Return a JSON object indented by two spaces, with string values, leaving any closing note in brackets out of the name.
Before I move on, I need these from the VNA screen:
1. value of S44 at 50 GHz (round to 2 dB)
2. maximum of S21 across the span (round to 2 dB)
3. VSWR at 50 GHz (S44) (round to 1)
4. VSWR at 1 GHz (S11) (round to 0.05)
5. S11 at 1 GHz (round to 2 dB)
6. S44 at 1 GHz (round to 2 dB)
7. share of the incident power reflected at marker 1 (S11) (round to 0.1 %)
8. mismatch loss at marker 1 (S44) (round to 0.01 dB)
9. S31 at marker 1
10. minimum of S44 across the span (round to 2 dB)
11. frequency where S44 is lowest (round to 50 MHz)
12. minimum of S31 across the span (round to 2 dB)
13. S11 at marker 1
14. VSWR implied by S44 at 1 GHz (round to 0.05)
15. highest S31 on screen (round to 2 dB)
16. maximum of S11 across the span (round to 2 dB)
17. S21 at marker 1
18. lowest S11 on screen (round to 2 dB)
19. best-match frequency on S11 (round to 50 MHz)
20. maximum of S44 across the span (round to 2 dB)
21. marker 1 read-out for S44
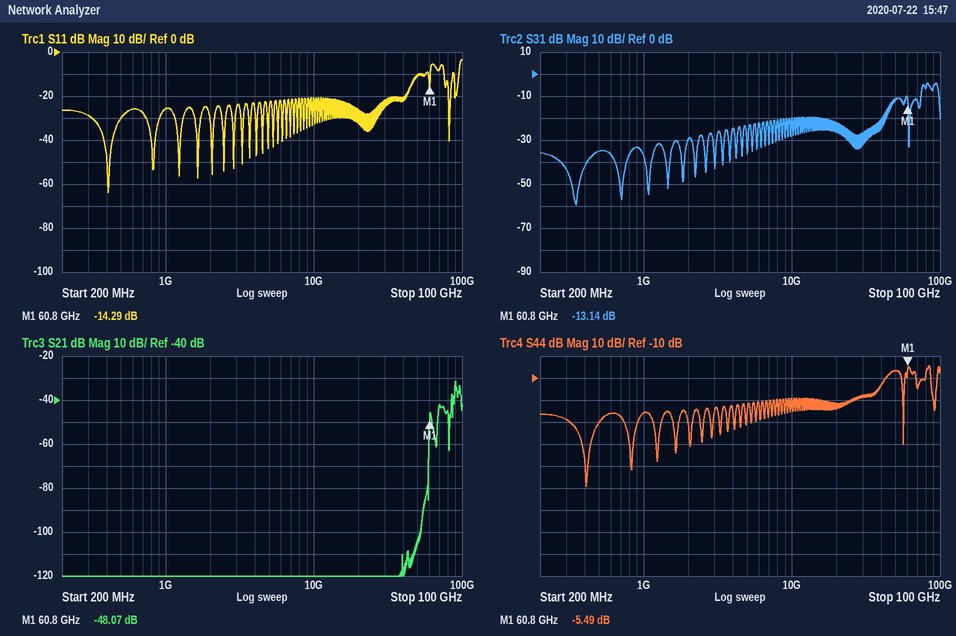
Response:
{
  "value of S44 at 50 GHz": "-6 dB",
  "maximum of S21 across the span": "-32 dB",
  "VSWR at 50 GHz (S44)": "3",
  "VSWR at 1 GHz (S11)": "1.10",
  "S11 at 1 GHz": "-26 dB",
  "S44 at 1 GHz": "-26 dB",
  "share of the incident power reflected at marker 1 (S11)": "3.7 %",
  "mismatch loss at marker 1 (S44)": "1.44 dB",
  "S31 at marker 1": "-13.14 dB",
  "minimum of S44 across the span": "-60 dB",
  "frequency where S44 is lowest": "400 MHz",
  "minimum of S31 across the span": "-60 dB",
  "S11 at marker 1": "-14.29 dB",
  "VSWR implied by S44 at 1 GHz": "1.10",
  "highest S31 on screen": "-4 dB",
  "maximum of S11 across the span": "-4 dB",
  "S21 at marker 1": "-48.07 dB",
  "lowest S11 on screen": "-64 dB",
  "best-match frequency on S11": "400 MHz",
  "maximum of S44 across the span": "-4 dB",
  "marker 1 read-out for S44": "-5.49 dB"
}
